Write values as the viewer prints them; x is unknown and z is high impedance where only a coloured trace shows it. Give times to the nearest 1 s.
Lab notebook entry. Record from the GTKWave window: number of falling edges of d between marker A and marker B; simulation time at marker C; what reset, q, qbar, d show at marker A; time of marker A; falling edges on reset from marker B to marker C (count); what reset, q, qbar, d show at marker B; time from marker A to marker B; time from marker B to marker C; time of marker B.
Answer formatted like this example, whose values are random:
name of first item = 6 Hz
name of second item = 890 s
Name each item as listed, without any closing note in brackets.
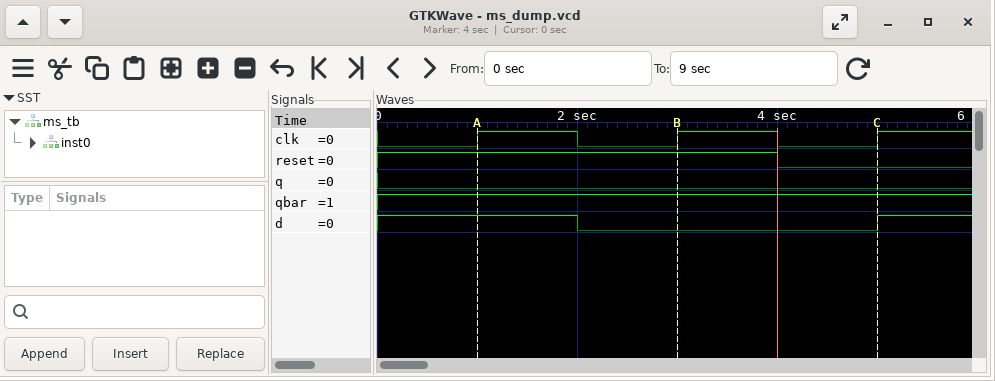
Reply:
number of falling edges of d between marker A and marker B = 1
simulation time at marker C = 5 s
what reset, q, qbar, d show at marker A = reset=1, q=0, qbar=1, d=1
time of marker A = 1 s
falling edges on reset from marker B to marker C = 1
what reset, q, qbar, d show at marker B = reset=1, q=0, qbar=1, d=0
time from marker A to marker B = 2 s
time from marker B to marker C = 2 s
time of marker B = 3 s
